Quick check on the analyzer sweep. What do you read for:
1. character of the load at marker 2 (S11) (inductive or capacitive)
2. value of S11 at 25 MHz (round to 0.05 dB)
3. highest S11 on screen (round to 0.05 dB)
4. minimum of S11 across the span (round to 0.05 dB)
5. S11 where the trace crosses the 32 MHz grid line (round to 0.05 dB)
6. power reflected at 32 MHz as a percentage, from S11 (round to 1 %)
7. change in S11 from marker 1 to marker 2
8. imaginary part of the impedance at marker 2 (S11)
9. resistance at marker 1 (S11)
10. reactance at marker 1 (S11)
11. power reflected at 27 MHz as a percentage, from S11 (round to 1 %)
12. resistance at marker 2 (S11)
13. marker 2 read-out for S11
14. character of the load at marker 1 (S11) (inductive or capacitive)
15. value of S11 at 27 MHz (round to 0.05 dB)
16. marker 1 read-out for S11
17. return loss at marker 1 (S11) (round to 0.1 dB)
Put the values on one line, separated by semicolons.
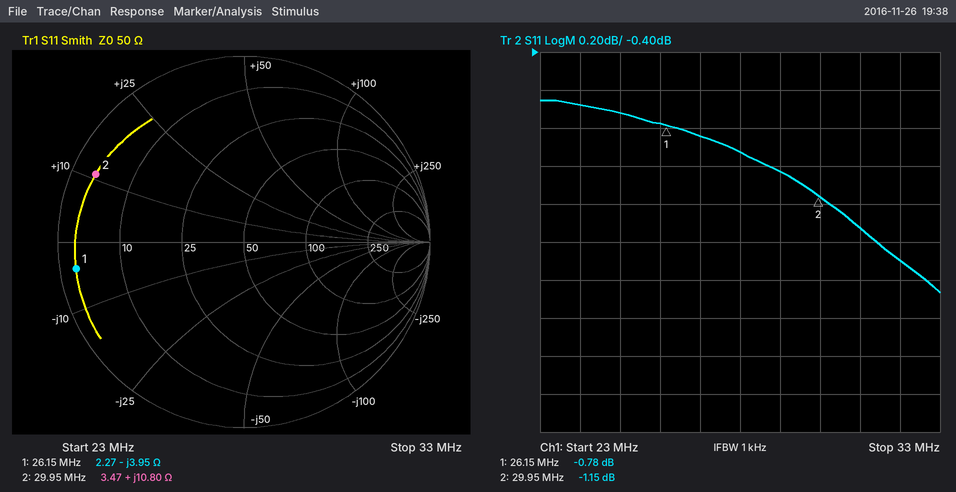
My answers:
inductive; -0.70 dB; -0.65 dB; -1.65 dB; -1.50 dB; 71 %; -0.37 dB; +10.80 Ω; 2.27 Ω; -3.95 Ω; 82 %; 3.47 Ω; -1.15 dB; capacitive; -0.85 dB; -0.78 dB; 0.8 dB
